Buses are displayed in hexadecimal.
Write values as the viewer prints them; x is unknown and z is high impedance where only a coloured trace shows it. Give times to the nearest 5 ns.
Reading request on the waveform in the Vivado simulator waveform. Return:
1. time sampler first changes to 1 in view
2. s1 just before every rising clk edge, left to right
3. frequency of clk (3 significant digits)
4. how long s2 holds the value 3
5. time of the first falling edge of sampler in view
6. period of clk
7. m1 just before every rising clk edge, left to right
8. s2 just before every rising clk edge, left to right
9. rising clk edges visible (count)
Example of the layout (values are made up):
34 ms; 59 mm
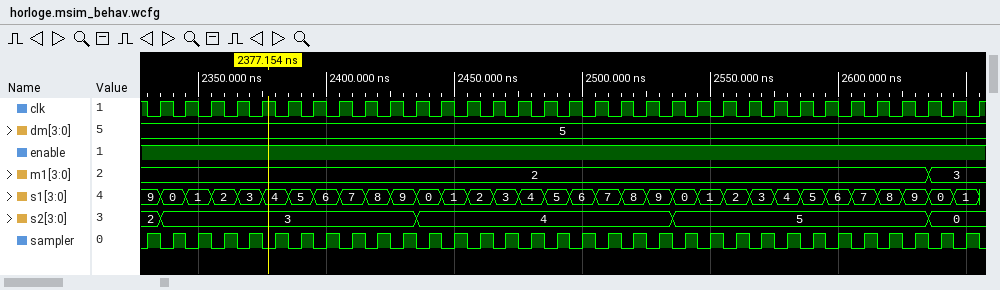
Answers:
2330 ns; 9, 0, 1, 2, 3, 4, 5, 6, 7, 8, 9, 0, 1, 2, 3, 4, 5, 6, 7, 8, 9, 0, 1, 2, 3, 4, 5, 6, 7, 8, 9, 0, 1; 100 MHz; 100 ns; 2335 ns; 10 ns; 2, 2, 2, 2, 2, 2, 2, 2, 2, 2, 2, 2, 2, 2, 2, 2, 2, 2, 2, 2, 2, 2, 2, 2, 2, 2, 2, 2, 2, 2, 2, 3, 3; 2, 3, 3, 3, 3, 3, 3, 3, 3, 3, 3, 4, 4, 4, 4, 4, 4, 4, 4, 4, 4, 5, 5, 5, 5, 5, 5, 5, 5, 5, 5, 0, 0; 33
